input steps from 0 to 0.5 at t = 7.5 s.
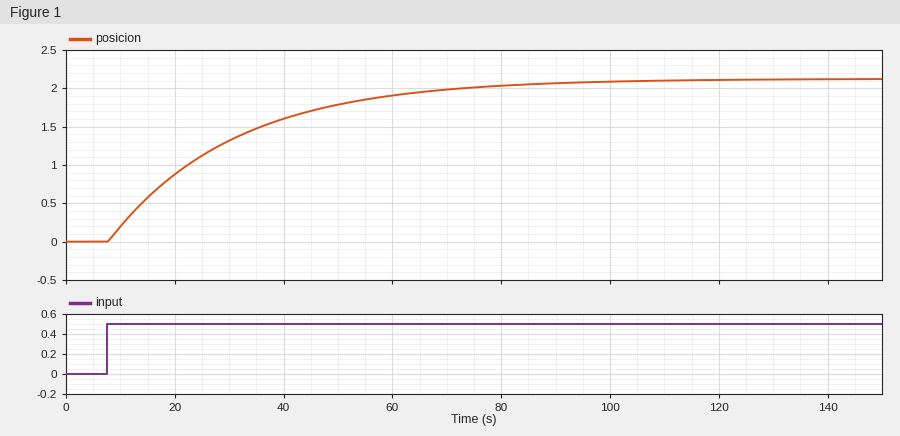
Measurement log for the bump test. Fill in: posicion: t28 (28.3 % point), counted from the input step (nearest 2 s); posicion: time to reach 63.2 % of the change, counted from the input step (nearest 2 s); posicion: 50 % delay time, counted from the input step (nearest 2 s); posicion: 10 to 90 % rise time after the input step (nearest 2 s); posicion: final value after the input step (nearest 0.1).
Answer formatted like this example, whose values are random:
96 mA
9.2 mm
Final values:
8 s
24 s
16 s
50 s
2.1
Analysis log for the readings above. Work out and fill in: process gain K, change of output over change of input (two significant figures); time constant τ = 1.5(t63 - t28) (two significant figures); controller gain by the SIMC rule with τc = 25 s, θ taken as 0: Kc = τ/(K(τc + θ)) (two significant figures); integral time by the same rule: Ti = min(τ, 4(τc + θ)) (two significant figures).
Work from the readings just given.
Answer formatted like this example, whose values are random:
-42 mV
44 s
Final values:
4.2
24 s
0.23
24 s
